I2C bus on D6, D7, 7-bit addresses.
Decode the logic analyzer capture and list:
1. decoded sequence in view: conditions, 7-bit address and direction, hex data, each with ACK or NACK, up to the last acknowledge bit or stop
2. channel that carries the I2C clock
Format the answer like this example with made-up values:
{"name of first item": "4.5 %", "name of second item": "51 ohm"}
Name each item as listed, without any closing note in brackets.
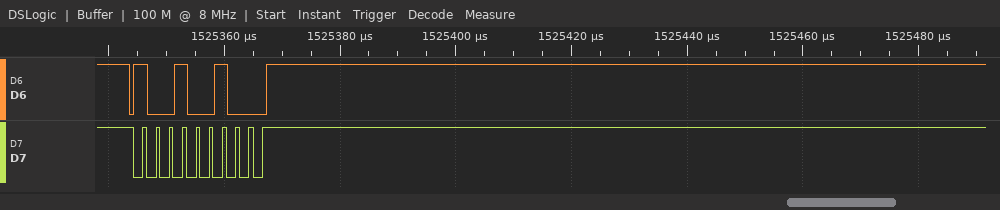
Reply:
{"decoded sequence in view: conditions, 7-bit address and direction, hex data, each with ACK or NACK, up to the last acknowledge bit or stop": "start, address 49 write ACK, stop", "channel that carries the I2C clock": "D7"}
